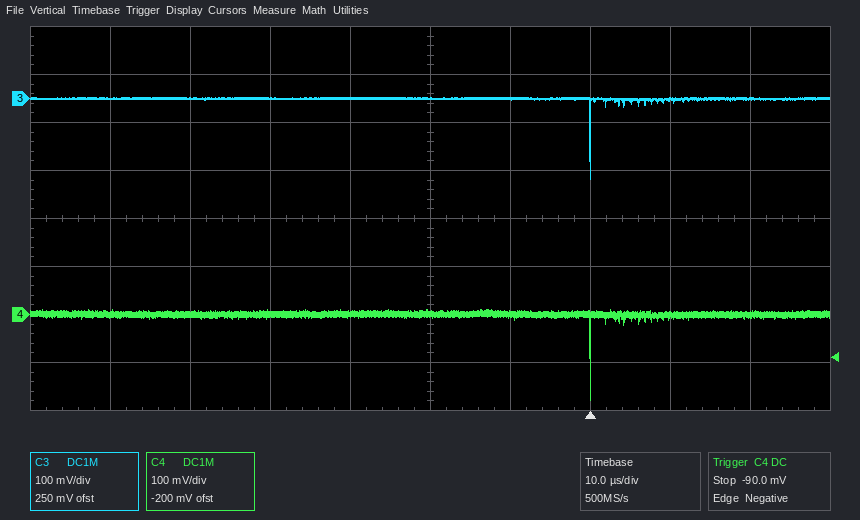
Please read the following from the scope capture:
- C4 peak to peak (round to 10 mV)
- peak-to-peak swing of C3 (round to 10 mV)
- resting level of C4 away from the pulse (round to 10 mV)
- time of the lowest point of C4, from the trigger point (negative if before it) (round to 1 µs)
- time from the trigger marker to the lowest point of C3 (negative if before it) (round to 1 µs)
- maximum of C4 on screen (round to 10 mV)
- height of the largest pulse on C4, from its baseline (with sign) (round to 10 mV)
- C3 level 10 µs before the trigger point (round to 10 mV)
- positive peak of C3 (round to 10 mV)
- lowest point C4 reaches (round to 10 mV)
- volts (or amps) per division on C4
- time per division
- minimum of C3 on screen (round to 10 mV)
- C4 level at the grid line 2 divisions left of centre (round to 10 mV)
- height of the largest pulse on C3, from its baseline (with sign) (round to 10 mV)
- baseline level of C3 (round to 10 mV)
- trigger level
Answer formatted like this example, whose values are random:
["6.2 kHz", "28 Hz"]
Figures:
["190 mV", "170 mV", "0 mV", "0 µs", "0 µs", "10 mV", "-180 mV", "0 mV", "0 mV", "-180 mV", "100 mV", "10 µs", "-170 mV", "0 mV", "-170 mV", "0 mV", "-90.0 mV"]
